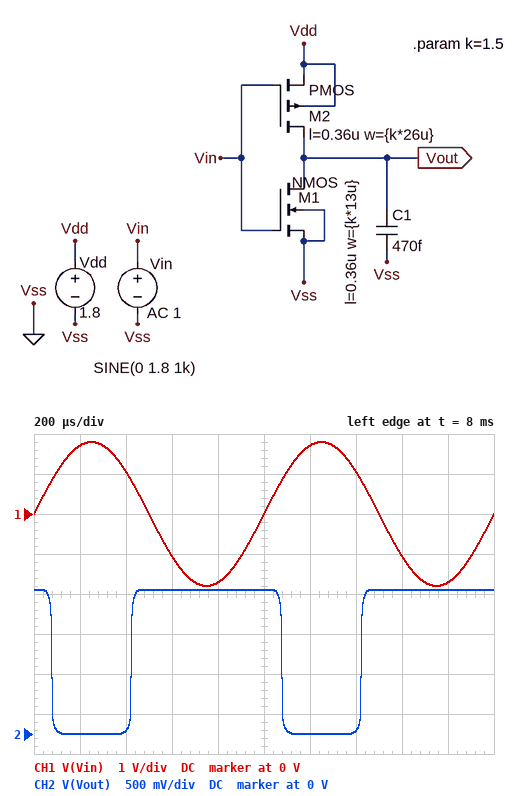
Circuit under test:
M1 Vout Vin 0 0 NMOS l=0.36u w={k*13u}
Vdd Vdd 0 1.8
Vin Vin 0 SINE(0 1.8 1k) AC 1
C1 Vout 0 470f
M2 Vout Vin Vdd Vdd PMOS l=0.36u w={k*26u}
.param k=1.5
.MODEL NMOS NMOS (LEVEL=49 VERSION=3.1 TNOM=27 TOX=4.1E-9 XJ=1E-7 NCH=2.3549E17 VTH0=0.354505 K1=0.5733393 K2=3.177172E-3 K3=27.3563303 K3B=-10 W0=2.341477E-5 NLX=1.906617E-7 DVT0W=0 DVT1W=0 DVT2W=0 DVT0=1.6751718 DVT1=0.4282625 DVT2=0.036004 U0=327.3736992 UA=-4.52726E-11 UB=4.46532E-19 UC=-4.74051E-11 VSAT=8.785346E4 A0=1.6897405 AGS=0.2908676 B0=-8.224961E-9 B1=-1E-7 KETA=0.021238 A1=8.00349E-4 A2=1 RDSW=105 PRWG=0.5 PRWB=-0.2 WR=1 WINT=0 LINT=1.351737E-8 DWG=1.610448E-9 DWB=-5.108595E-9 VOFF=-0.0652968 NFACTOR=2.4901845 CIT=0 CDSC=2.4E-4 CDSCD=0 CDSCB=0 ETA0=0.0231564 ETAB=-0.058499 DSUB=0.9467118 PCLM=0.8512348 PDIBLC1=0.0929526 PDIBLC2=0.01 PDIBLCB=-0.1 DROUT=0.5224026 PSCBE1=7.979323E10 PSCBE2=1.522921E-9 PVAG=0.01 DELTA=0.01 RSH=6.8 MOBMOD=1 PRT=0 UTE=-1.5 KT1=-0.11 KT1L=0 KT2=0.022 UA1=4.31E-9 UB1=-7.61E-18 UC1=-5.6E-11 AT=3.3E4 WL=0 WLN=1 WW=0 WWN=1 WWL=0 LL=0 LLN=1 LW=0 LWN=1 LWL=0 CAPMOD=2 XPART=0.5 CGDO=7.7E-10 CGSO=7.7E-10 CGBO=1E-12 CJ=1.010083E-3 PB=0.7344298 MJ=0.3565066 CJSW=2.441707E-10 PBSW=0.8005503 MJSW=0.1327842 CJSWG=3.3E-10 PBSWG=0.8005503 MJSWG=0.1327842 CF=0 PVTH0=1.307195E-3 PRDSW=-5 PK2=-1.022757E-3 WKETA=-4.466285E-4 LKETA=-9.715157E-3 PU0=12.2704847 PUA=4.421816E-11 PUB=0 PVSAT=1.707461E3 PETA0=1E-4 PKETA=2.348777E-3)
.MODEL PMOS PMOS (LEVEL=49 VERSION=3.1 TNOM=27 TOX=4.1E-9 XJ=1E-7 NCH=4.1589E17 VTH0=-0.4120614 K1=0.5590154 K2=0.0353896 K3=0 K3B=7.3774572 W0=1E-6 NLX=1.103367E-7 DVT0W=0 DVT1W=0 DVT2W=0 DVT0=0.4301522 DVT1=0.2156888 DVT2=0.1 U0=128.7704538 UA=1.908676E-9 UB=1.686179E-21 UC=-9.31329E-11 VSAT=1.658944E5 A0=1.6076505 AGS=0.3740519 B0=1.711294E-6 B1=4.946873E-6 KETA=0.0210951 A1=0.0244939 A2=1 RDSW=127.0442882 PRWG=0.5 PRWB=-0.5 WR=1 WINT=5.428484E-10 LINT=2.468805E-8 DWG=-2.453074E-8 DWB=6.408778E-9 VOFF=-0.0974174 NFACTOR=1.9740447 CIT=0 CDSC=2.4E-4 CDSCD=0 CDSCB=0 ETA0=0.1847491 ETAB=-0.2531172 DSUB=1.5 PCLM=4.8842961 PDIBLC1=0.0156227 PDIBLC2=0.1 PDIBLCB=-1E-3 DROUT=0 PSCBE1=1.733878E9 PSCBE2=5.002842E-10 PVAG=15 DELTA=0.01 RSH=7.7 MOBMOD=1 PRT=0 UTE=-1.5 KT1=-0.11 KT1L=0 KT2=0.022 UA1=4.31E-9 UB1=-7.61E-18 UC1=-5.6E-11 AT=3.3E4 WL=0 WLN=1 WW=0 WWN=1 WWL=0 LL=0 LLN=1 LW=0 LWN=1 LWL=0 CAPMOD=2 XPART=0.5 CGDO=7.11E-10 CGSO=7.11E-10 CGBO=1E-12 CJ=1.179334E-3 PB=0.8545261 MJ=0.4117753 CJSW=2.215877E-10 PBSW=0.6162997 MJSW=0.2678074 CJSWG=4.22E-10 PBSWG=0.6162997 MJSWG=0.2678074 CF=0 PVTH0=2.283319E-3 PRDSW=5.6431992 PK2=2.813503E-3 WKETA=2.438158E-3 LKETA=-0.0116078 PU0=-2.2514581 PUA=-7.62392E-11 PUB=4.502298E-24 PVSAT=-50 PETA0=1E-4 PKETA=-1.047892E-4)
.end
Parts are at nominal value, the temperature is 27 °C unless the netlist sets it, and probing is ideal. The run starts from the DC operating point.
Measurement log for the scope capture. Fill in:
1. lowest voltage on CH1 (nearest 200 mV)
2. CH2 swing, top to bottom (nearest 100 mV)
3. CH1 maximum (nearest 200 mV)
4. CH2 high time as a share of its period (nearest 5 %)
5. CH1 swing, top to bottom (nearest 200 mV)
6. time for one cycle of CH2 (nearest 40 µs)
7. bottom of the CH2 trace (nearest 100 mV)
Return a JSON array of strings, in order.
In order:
["-1.8 V", "1.8 V", "1.8 V", "65 %", "3.6 V", "1.00 ms", "0 V"]
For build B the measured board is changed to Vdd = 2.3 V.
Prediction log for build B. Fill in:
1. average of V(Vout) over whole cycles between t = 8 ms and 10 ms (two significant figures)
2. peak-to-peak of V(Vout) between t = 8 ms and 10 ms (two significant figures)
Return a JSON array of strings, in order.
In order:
["1.6 V", "2.3 V"]
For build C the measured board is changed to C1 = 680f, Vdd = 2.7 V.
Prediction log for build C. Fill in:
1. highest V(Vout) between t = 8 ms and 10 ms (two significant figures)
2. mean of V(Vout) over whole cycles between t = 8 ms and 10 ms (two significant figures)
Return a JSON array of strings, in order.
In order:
["2.7 V", "2.0 V"]
